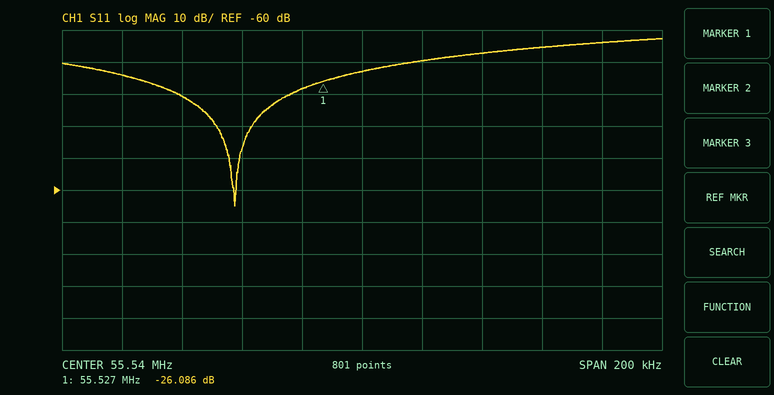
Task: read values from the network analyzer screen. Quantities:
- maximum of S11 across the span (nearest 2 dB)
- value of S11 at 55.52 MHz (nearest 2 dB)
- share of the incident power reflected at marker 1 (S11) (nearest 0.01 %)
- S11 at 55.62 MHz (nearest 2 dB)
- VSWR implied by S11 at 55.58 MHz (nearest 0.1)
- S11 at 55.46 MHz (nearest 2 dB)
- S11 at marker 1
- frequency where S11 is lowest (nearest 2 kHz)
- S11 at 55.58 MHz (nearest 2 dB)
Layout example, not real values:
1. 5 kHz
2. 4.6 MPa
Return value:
1. -12 dB
2. -28 dB
3. 0.25 %
4. -14 dB
5. 1.3
6. -24 dB
7. -26.086 dB
8. 55.498 MHz
9. -18 dB
